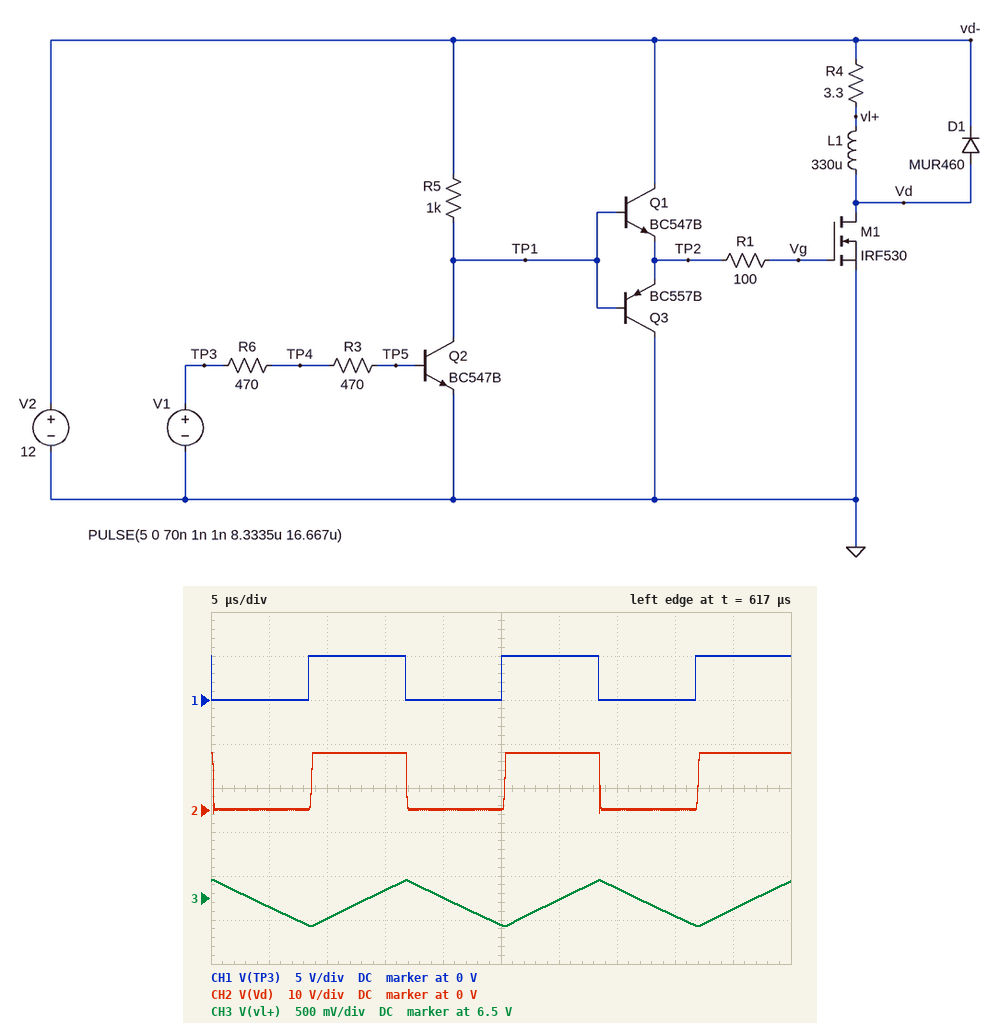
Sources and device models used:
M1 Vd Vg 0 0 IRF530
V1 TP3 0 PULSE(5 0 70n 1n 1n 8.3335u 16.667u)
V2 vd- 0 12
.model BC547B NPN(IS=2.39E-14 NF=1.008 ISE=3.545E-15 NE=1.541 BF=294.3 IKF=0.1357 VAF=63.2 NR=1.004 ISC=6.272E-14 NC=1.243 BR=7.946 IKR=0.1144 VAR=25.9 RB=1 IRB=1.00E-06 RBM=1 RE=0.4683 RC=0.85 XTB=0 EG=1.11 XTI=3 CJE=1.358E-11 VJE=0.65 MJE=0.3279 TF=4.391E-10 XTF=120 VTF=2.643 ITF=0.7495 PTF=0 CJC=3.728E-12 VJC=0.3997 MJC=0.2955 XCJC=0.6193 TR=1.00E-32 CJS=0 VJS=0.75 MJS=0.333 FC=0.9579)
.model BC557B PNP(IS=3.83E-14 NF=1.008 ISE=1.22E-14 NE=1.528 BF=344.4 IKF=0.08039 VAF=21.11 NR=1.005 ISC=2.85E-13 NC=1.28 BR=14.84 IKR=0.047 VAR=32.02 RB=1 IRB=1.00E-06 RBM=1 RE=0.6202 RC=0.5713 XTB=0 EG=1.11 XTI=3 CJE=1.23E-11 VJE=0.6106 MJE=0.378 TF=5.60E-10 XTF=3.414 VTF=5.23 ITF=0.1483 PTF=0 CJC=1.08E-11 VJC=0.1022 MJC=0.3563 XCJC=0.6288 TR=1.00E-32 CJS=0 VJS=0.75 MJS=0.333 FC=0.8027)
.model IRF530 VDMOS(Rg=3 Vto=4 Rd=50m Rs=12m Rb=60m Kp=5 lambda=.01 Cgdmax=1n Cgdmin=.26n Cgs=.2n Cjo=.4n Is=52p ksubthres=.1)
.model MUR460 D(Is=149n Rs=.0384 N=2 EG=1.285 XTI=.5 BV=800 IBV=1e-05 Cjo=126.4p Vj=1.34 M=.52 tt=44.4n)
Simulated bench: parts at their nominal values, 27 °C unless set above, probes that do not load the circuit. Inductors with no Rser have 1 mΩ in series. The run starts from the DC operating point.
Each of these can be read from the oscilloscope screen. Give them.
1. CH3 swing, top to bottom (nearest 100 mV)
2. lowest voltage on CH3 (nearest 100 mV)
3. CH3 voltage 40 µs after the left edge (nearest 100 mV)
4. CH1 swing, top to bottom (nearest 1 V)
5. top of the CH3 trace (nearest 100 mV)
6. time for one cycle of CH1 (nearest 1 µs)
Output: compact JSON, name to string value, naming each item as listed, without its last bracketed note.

{"CH3 swing, top to bottom": "500 mV", "lowest voltage on CH3": "6.2 V", "CH3 voltage 40 µs after the left edge": "6.3 V", "CH1 swing, top to bottom": "5 V", "top of the CH3 trace": "6.7 V", "time for one cycle of CH1": "17 µs"}
